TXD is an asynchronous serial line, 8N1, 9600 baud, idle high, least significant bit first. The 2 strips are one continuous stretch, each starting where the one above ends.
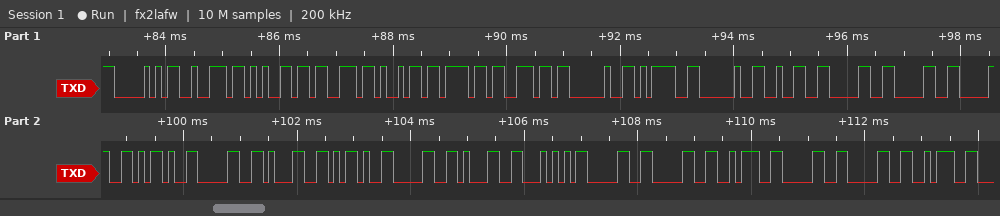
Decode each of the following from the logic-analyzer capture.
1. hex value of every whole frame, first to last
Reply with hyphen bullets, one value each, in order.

- 50 72 65 73 69 6F 6E 20 3D 20 32 30 30 30 2D 30 31 2D 30 31 54 30 30 3A 30 30 3A
